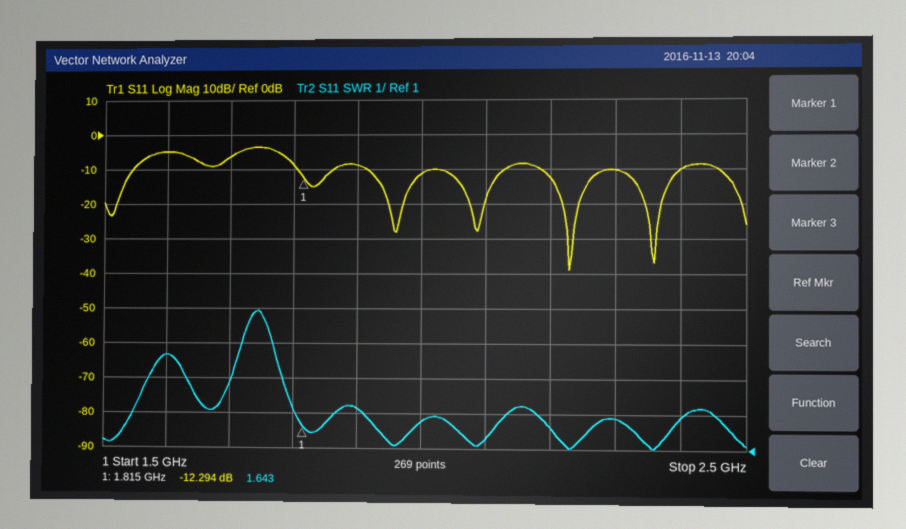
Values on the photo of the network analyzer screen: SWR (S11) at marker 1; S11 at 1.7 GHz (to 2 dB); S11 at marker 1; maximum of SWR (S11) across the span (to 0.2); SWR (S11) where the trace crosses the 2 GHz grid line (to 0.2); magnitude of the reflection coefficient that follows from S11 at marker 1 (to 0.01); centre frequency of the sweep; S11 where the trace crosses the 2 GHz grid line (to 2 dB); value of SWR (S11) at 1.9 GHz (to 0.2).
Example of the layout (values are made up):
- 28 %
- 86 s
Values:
- 1.643
- -6 dB
- -12.294 dB
- 5.0
- 1.8
- 0.24
- 2 GHz
- -12 dB
- 2.2
